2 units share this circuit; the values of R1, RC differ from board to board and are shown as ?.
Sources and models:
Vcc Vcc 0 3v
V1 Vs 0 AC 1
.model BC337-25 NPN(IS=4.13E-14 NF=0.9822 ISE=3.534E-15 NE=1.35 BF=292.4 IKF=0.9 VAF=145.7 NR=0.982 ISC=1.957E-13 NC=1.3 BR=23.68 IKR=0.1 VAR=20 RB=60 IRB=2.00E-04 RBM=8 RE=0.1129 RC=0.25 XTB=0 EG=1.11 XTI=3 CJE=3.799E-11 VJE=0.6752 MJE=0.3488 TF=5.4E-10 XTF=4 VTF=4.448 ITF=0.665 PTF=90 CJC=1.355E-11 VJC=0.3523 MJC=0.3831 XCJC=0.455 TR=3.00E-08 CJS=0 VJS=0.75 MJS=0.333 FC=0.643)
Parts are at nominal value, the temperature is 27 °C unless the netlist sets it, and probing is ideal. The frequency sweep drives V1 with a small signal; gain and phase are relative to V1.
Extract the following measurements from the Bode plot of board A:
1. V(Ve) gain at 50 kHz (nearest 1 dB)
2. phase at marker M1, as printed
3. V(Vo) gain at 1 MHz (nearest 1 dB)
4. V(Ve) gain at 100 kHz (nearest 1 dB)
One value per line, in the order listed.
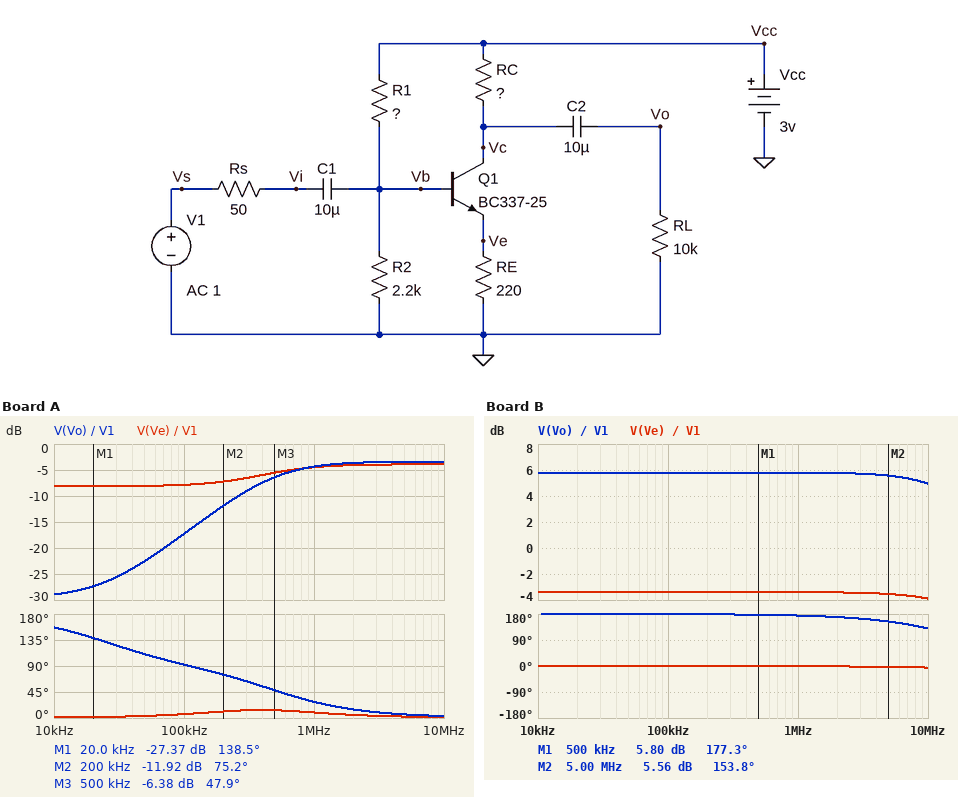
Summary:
-8 dB
138.5 deg
-4 dB
-8 dB
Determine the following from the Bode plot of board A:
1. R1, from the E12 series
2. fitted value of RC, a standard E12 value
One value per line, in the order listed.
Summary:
4.7 kΩ
2.7 kΩ
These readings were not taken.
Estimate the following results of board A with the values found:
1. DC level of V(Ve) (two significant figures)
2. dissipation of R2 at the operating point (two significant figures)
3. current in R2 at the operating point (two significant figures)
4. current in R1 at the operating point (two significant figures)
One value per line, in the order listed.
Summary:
240 mV
340 µW
390 µA
450 µA
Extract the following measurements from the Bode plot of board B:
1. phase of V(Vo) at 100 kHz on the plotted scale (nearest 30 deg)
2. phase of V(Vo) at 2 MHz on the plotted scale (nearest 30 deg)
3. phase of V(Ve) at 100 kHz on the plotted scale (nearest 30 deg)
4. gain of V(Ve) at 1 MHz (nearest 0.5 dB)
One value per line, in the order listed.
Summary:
180 deg
180 deg
0 deg
-3.5 dB
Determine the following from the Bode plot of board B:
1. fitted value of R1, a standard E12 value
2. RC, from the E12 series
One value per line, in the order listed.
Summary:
8.2 kΩ
680 Ω
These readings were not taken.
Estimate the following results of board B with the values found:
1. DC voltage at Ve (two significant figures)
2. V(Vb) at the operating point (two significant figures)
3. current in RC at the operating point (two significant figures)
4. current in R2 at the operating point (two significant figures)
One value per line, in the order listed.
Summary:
59 mV
630 mV
270 µA
290 µA
